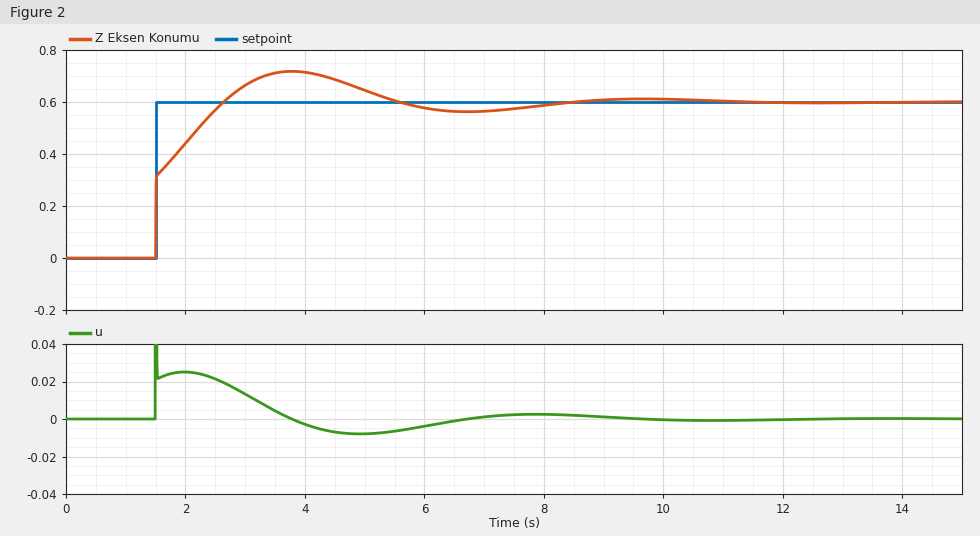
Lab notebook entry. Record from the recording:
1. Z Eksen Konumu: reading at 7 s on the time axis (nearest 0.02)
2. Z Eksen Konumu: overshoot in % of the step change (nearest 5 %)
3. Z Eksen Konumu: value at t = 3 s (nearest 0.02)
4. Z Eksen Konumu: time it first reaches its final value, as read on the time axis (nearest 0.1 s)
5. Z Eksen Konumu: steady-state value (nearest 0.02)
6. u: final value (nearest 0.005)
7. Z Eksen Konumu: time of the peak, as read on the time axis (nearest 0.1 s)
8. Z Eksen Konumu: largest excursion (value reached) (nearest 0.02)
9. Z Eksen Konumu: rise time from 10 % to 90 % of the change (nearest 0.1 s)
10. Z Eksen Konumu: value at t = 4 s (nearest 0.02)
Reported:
0.56
20 %
0.66
2.6 s
0.60
0.000
3.8 s
0.72
0.9 s
0.72
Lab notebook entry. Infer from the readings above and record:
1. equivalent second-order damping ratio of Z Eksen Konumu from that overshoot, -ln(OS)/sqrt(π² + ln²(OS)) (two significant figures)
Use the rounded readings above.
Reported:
0.46
